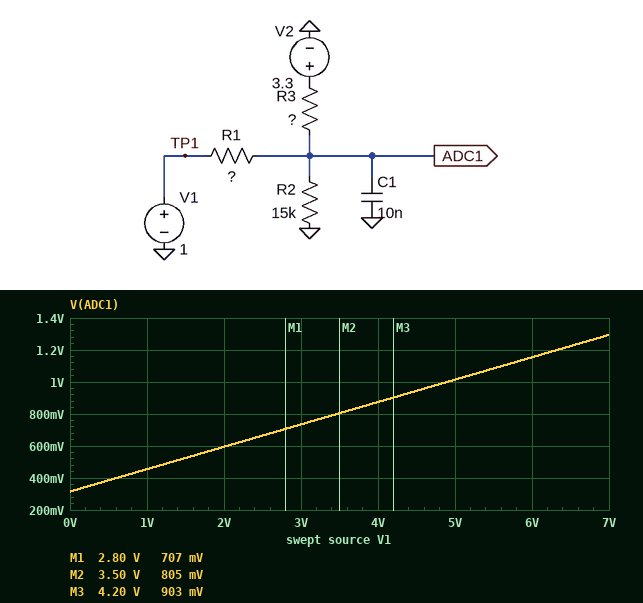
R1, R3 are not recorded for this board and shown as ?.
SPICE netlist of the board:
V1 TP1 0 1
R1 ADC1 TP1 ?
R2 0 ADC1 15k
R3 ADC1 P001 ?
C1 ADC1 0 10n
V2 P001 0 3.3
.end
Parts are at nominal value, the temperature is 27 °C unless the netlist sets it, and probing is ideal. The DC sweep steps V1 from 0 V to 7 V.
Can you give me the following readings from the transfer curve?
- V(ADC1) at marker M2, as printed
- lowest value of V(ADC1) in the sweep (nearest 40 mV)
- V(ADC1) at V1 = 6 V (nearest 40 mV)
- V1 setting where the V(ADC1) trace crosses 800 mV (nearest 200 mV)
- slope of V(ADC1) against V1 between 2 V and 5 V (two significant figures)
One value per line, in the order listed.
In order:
805 mV
320 mV
1.16 V
3.4 V
0.14 V/V
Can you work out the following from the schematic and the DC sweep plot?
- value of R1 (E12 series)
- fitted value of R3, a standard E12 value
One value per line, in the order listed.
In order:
82 kΩ
120 kΩ
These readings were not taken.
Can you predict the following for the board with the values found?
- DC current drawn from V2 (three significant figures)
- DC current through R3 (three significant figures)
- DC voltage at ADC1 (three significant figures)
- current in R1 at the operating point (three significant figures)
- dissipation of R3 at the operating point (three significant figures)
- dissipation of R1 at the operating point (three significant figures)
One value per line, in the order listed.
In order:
23.7 µA
23.7 µA
455 mV
6.64 µA
67.4 µW
3.62 µW
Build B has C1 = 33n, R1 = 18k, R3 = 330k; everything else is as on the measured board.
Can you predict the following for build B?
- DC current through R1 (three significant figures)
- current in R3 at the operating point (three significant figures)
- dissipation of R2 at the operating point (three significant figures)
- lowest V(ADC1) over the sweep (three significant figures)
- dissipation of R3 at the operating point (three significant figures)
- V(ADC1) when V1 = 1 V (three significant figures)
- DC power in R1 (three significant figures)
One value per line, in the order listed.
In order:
26.5 µA
8.41 µA
18.3 µW
79.8 mV
23.4 µW
523 mV
12.6 µW
